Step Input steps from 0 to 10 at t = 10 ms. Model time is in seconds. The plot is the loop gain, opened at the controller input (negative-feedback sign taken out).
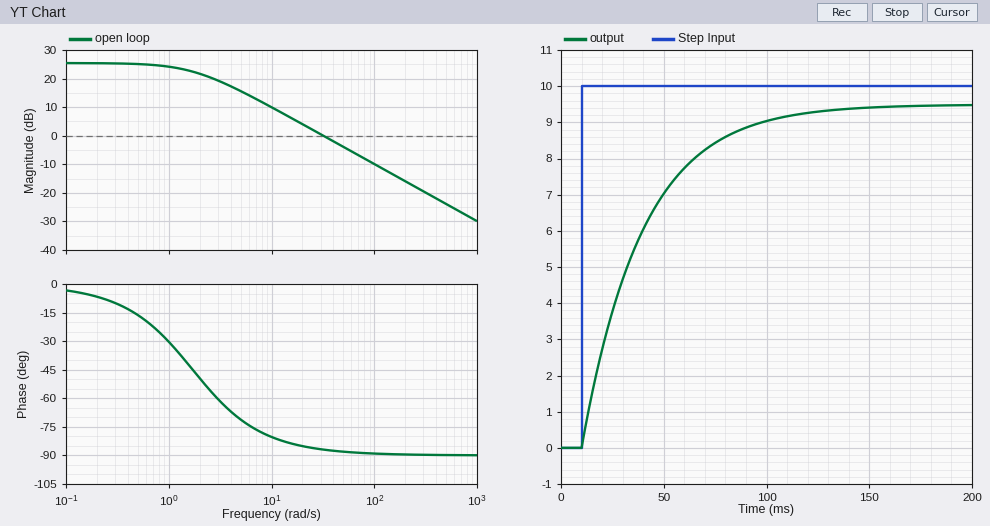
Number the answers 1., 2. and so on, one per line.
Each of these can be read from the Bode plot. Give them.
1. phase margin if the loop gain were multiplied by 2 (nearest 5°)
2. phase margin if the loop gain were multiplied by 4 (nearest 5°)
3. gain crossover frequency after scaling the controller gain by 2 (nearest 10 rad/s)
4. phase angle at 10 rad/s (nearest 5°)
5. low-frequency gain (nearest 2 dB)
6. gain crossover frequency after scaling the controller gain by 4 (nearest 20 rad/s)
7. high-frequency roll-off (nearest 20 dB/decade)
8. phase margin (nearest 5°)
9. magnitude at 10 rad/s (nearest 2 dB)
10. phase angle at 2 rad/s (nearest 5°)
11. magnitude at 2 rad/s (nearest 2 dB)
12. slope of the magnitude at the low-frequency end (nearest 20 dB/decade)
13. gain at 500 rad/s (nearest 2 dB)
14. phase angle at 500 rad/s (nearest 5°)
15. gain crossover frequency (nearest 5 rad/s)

1. 90°
2. 90°
3. 60 rad/s
4. -80°
5. 26 dB
6. 120 rad/s
7. -20 dB/decade
8. 95°
9. 10 dB
10. -50°
11. 22 dB
12. 0 dB/decade
13. -24 dB
14. -90°
15. 30 rad/s
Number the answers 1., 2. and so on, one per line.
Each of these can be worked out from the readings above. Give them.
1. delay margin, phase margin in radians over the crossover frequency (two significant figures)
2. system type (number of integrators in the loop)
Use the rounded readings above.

1. 0.055 s
2. 0
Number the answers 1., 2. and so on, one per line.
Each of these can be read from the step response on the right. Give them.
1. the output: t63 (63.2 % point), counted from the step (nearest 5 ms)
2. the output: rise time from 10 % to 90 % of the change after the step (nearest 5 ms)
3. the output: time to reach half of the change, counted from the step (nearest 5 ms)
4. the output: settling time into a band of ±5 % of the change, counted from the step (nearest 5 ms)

1. 30 ms
2. 65 ms
3. 20 ms
4. 90 ms
